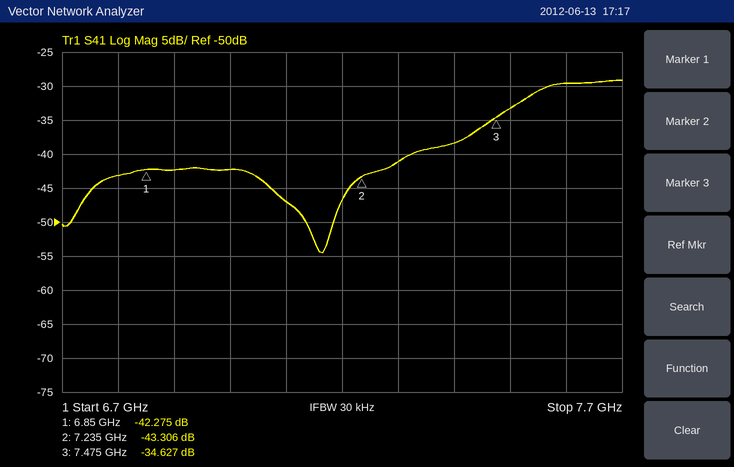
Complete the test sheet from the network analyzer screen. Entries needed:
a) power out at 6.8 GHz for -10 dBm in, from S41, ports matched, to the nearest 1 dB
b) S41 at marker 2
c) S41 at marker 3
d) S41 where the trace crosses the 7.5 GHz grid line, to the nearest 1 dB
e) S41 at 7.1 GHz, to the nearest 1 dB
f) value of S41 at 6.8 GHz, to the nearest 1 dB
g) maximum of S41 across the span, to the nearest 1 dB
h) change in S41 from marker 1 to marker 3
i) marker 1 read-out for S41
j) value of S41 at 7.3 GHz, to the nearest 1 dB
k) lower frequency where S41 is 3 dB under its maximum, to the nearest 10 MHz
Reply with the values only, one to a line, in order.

-53 dBm
-43.306 dB
-34.627 dB
-33 dB
-47 dB
-43 dB
-29 dB
7.648 dB
-42.275 dB
-41 dB
7.52 GHz
